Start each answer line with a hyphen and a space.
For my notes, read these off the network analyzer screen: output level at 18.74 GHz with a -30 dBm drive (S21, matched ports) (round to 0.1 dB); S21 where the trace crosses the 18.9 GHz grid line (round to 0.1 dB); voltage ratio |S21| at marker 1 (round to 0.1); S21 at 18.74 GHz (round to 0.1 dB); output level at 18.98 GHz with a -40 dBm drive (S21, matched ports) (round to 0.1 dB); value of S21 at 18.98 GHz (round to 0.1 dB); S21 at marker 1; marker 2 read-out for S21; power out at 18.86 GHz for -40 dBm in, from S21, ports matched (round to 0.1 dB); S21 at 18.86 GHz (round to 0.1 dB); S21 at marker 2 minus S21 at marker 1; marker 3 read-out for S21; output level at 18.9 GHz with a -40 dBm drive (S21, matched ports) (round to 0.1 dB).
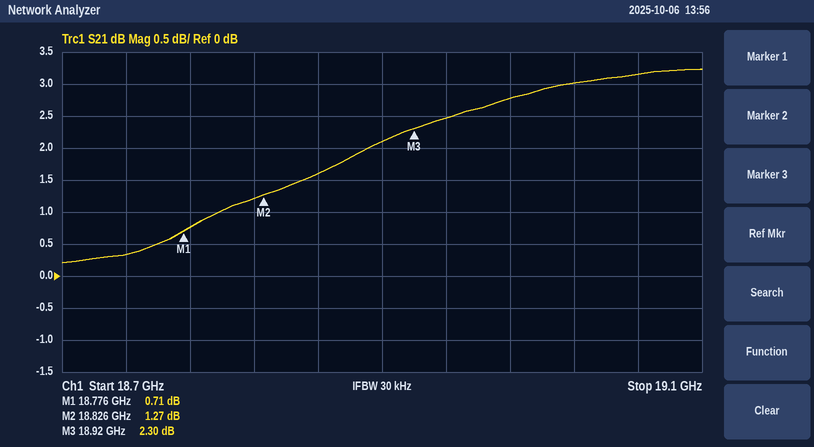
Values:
- -29.7 dBm
- 2.1 dB
- 1.1
- 0.3 dB
- -37.2 dBm
- 2.8 dB
- 0.71 dB
- 1.27 dB
- -38.4 dBm
- 1.6 dB
- 0.56 dB
- 2.30 dB
- -37.9 dBm
